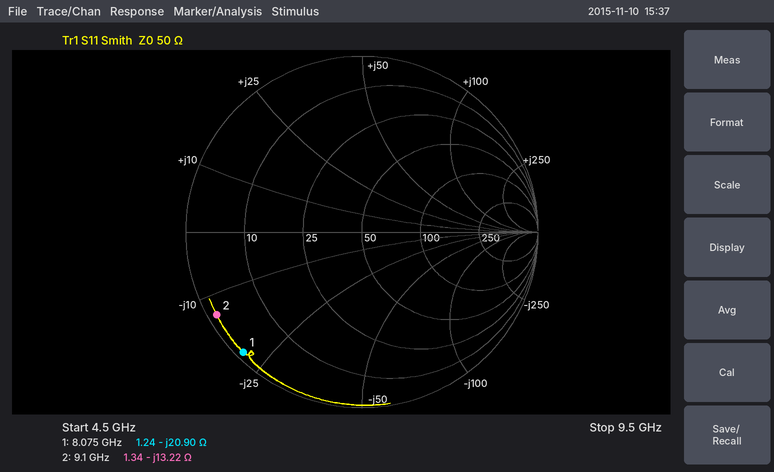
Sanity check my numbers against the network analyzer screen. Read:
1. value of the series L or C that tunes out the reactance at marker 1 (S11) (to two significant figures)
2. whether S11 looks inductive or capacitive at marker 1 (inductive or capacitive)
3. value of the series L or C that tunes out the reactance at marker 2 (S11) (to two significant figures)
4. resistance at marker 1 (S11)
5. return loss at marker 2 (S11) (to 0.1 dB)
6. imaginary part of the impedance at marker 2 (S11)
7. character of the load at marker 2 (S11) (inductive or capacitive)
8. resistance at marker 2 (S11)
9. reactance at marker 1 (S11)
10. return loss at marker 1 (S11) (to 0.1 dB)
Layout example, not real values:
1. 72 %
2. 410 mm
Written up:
1. 410 pH
2. capacitive
3. 230 pH
4. 1.24 Ω
5. 0.4 dB
6. -13.22 Ω
7. capacitive
8. 1.34 Ω
9. -20.90 Ω
10. 0.4 dB
